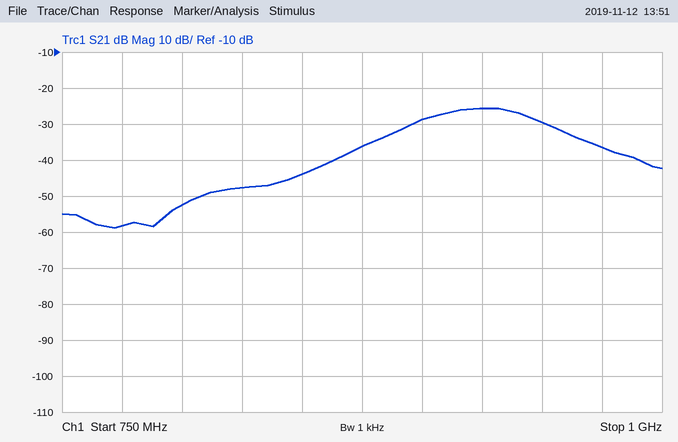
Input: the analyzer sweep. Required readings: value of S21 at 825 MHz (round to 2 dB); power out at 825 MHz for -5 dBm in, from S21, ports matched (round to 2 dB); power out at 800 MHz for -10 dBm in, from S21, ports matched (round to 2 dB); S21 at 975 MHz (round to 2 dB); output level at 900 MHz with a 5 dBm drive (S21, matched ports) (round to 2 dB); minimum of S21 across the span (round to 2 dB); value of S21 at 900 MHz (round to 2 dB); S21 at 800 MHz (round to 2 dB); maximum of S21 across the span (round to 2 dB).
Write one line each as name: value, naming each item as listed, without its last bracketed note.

value of S21 at 825 MHz: -48 dB
power out at 825 MHz for -5 dBm in, from S21, ports matched: -52 dBm
power out at 800 MHz for -10 dBm in, from S21, ports matched: -62 dBm
S21 at 975 MHz: -36 dB
output level at 900 MHz with a 5 dBm drive (S21, matched ports): -24 dBm
minimum of S21 across the span: -58 dB
value of S21 at 900 MHz: -28 dB
S21 at 800 MHz: -52 dB
maximum of S21 across the span: -26 dB
